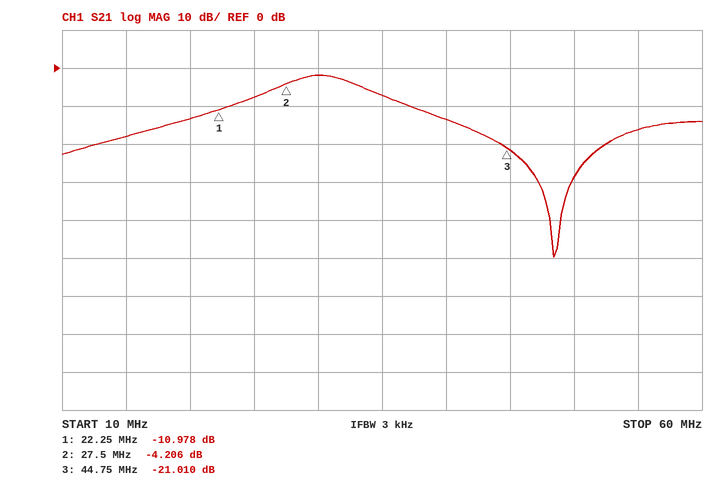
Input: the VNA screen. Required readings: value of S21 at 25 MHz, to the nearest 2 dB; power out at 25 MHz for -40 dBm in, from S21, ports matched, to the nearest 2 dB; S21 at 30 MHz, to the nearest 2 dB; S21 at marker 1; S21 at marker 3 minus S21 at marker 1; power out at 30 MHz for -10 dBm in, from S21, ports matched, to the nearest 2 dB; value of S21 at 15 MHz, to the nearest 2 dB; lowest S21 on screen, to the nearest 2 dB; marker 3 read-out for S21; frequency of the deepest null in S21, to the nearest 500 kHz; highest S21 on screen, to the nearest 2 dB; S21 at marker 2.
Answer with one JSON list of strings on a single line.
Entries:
["-8 dB", "-48 dBm", "-2 dB", "-10.978 dB", "-10.032 dB", "-12 dBm", "-18 dB", "-50 dB", "-21.010 dB", "48.5 MHz", "-2 dB", "-4.206 dB"]
